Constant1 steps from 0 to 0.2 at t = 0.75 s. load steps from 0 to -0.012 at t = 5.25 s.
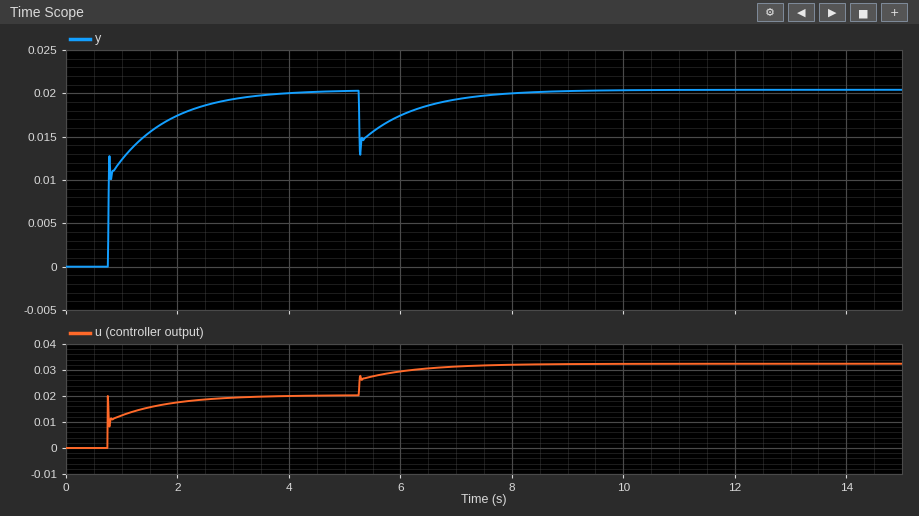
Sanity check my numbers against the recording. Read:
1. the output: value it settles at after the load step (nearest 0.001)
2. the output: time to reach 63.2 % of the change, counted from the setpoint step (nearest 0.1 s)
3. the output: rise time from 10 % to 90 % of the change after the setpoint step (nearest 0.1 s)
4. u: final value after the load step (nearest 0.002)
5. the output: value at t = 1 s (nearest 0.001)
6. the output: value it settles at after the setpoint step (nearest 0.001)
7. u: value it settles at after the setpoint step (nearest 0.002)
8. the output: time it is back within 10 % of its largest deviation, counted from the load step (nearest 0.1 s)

0.020
0.3 s
1.6 s
0.032
0.012
0.020
0.020
2.2 s
